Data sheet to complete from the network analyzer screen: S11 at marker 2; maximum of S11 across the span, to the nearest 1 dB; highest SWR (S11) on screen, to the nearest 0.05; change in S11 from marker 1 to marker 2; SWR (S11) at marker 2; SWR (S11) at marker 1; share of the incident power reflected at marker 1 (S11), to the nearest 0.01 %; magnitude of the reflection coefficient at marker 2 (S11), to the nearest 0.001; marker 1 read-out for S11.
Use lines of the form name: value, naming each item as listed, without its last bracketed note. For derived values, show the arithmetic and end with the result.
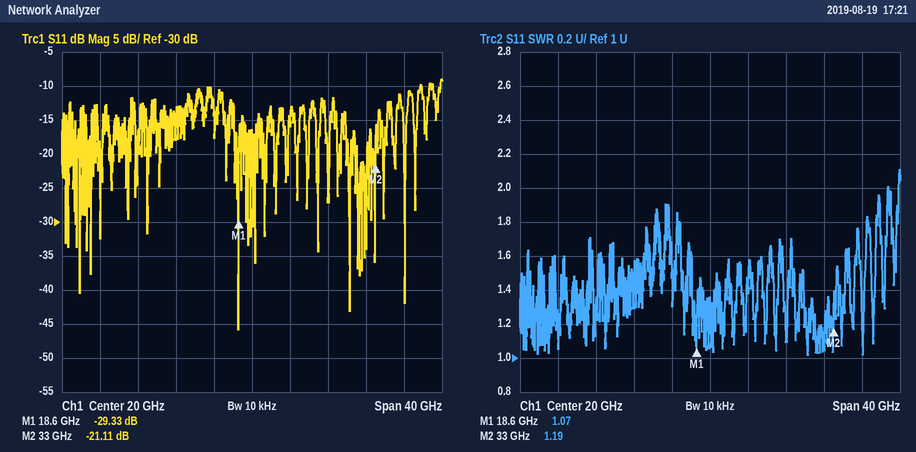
S11 at marker 2: -21.11 dB
maximum of S11 across the span, to the nearest 1 dB: -9 dB
highest SWR (S11) on screen, to the nearest 0.05: 2.10
change in S11 from marker 1 to marker 2: -21.11 − (-29.33) = 8.22 dB
SWR (S11) at marker 2: 1.19
SWR (S11) at marker 1: 1.07
share of the incident power reflected at marker 1 (S11), to the nearest 0.01 %: 10^(-29.33/10) ≈ 0.12 %
magnitude of the reflection coefficient at marker 2 (S11), to the nearest 0.001: 10^(-21.11/20) ≈ 0.088
marker 1 read-out for S11: -29.33 dB
